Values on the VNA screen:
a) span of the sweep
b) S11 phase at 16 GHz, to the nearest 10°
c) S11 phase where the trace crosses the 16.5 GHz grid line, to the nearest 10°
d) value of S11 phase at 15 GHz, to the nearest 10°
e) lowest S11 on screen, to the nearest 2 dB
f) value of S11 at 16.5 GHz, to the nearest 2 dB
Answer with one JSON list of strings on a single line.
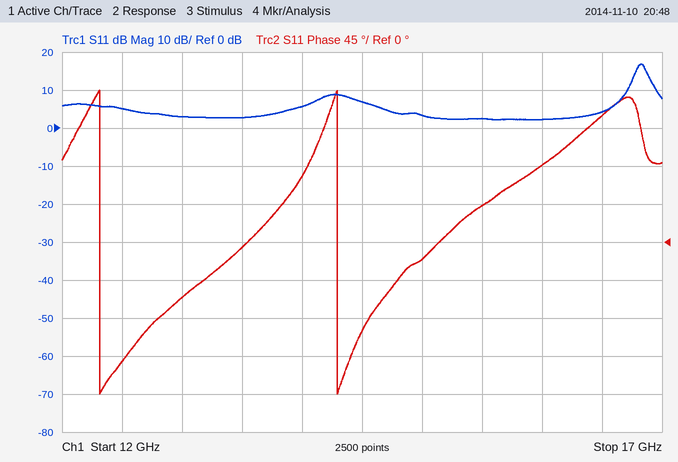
["5 GHz", "90°", "150°", "-20°", "2 dB", "4 dB"]
